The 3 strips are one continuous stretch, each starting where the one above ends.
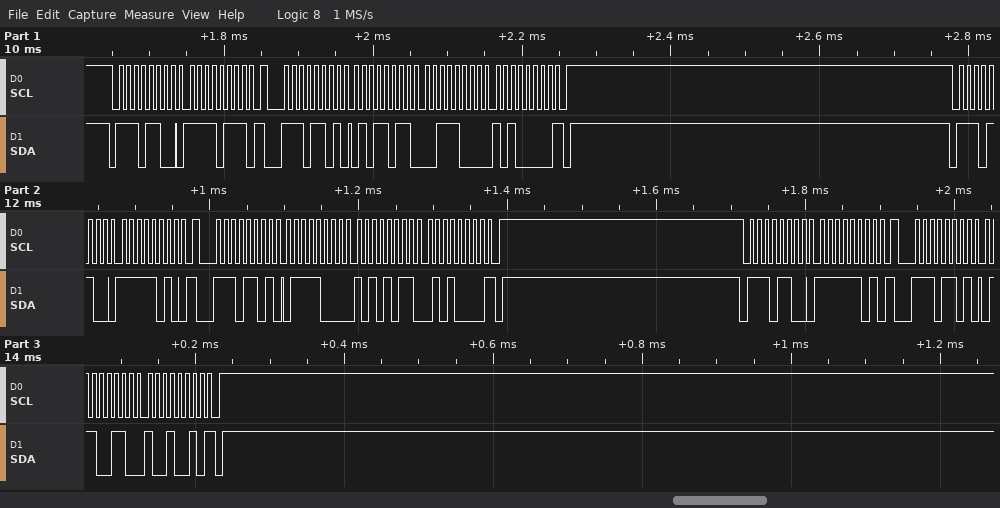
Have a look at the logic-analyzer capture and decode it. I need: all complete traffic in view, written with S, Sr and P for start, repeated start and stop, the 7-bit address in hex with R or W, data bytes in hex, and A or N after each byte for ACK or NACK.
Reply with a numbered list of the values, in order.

1. S 76W A F7 A Sr 76R A 5B A 38 A A0 N P S 76W A FA A Sr 76R A 78 A AB A 50 N P S 76W A FD A Sr 76R A 66 A 92 N P
